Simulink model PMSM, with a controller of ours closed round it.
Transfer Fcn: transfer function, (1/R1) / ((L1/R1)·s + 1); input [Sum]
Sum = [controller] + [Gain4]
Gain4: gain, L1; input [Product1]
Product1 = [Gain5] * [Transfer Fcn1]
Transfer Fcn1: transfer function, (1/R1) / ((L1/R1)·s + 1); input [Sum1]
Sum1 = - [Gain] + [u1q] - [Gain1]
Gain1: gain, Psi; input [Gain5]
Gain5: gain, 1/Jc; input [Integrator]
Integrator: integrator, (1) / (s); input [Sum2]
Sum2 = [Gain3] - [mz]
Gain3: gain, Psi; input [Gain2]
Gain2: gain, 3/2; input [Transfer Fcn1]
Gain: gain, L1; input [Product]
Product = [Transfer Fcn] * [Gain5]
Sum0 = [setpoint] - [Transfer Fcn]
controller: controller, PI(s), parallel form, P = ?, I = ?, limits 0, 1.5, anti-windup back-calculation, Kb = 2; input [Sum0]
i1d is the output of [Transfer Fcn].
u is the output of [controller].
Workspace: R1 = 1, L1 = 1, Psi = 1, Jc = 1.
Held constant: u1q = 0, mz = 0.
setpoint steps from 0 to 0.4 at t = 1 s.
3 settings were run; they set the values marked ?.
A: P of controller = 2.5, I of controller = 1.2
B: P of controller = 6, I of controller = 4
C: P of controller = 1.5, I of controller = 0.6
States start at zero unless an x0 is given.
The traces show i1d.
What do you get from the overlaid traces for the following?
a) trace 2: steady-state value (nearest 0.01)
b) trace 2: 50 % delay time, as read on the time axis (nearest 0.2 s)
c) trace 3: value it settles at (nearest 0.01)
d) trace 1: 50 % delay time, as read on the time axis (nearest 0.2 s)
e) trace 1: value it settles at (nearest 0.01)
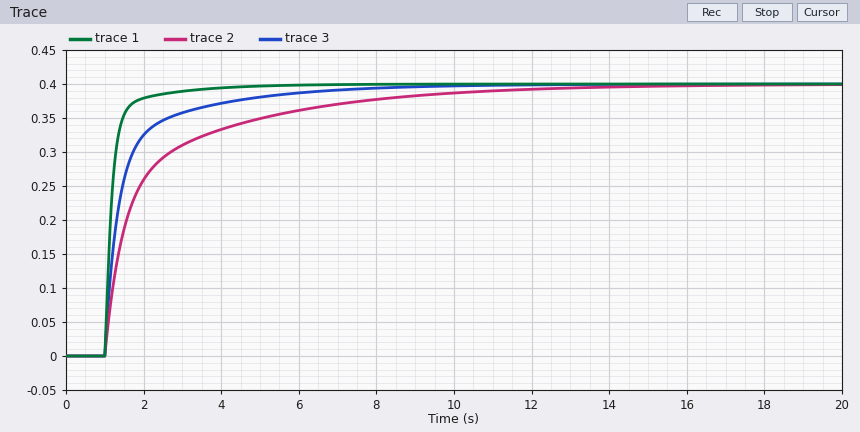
0.40
1.6 s
0.40
1.2 s
0.40
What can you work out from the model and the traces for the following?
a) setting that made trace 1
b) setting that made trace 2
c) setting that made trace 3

B
C
A
